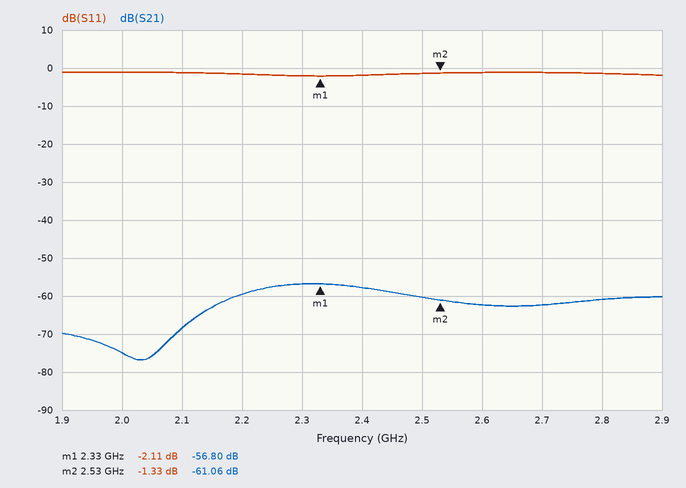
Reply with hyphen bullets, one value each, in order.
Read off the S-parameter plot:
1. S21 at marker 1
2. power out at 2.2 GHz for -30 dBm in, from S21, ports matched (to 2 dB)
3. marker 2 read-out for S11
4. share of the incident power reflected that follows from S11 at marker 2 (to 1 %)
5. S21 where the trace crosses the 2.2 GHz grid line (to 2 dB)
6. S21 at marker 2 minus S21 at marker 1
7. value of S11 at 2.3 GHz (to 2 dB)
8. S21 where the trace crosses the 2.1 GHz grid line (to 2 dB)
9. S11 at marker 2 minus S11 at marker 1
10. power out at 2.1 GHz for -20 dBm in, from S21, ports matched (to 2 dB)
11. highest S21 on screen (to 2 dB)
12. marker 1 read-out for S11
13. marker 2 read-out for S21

- -56.80 dB
- -90 dBm
- -1.33 dB
- 74 %
- -60 dB
- -4.26 dB
- -2 dB
- -68 dB
- 0.78 dB
- -88 dBm
- -56 dB
- -2.11 dB
- -61.06 dB
